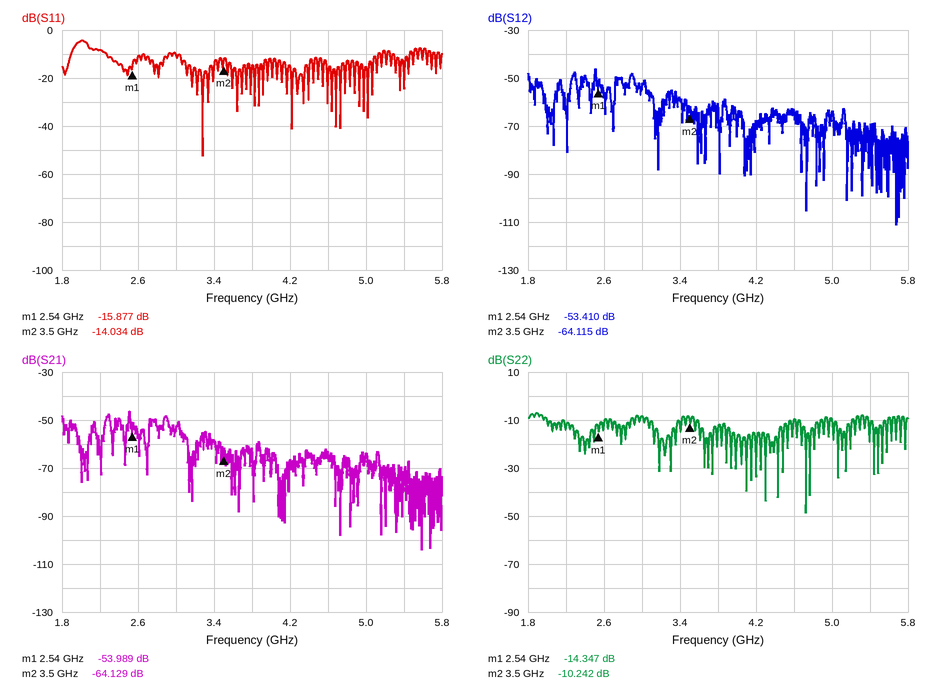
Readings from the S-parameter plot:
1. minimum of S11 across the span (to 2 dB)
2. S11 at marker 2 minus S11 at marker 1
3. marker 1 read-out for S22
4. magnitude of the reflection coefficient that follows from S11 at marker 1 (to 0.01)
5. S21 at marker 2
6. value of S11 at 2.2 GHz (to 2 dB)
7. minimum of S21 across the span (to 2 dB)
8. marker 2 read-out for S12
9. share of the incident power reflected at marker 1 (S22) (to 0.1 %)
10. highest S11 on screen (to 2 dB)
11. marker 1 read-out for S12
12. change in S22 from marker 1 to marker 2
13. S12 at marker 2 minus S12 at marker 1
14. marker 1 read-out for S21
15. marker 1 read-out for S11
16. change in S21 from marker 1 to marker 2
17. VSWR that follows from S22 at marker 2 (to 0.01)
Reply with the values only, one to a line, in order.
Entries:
-52 dB
1.843 dB
-14.347 dB
0.16
-64.129 dB
-8 dB
-104 dB
-64.115 dB
3.7 %
-4 dB
-53.410 dB
4.105 dB
-10.705 dB
-53.989 dB
-15.877 dB
-10.140 dB
1.89
